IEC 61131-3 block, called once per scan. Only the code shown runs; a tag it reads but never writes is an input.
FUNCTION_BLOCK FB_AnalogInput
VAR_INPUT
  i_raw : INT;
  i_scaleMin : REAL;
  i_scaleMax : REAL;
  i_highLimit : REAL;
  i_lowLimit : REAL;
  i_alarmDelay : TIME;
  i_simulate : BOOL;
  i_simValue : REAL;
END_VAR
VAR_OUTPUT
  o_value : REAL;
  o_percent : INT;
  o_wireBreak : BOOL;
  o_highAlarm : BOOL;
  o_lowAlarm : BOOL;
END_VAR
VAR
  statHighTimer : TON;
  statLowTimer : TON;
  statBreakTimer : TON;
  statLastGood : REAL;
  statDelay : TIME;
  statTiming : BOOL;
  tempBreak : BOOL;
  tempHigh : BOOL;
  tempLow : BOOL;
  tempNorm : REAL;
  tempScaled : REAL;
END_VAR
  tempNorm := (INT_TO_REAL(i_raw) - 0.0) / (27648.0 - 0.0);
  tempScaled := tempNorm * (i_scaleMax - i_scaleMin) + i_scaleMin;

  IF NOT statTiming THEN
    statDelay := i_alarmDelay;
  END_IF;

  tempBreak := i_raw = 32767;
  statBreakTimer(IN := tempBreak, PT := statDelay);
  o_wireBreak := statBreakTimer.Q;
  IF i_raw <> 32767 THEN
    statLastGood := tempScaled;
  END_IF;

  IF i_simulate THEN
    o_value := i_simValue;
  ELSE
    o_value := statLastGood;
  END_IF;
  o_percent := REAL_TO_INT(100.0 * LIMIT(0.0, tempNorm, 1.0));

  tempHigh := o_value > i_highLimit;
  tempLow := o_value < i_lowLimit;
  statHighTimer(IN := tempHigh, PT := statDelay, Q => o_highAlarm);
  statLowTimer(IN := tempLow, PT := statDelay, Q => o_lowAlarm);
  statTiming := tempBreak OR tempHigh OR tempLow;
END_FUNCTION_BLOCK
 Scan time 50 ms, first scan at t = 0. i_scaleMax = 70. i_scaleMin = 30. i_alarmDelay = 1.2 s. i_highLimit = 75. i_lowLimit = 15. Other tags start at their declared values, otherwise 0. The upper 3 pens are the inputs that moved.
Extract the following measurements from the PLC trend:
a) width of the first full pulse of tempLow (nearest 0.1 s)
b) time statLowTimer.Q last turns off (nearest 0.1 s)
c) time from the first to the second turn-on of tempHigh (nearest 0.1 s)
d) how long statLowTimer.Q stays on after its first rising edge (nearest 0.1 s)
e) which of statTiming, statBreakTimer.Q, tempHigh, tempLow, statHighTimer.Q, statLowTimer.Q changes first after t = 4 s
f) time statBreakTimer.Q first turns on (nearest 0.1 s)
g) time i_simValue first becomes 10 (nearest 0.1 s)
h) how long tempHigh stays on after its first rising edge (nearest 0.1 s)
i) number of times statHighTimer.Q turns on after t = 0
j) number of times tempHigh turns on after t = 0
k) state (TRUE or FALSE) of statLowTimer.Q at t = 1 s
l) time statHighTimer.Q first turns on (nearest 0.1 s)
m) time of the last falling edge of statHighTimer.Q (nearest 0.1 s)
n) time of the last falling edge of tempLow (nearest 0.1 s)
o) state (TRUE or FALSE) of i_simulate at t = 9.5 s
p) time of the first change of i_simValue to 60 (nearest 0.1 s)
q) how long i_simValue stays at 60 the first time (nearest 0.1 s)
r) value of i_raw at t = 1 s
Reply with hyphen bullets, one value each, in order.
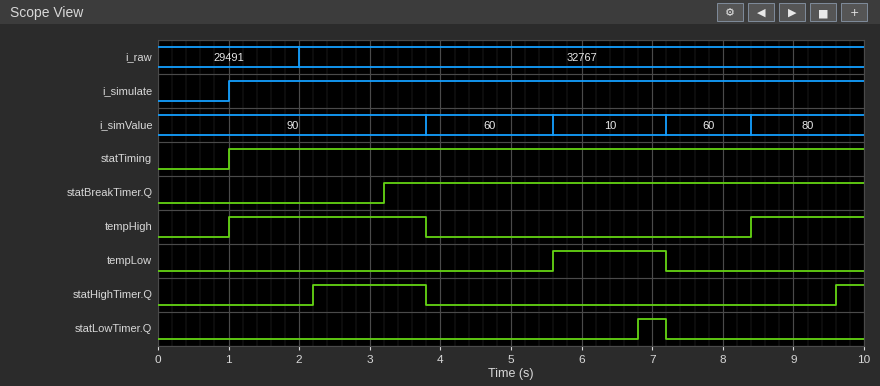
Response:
- 1.6 s
- 7.2 s
- 7.4 s
- 0.4 s
- tempLow
- 3.2 s
- 5.6 s
- 2.8 s
- 2
- 2
- FALSE
- 2.2 s
- 3.8 s
- 7.2 s
- TRUE
- 3.8 s
- 1.8 s
- 29491
